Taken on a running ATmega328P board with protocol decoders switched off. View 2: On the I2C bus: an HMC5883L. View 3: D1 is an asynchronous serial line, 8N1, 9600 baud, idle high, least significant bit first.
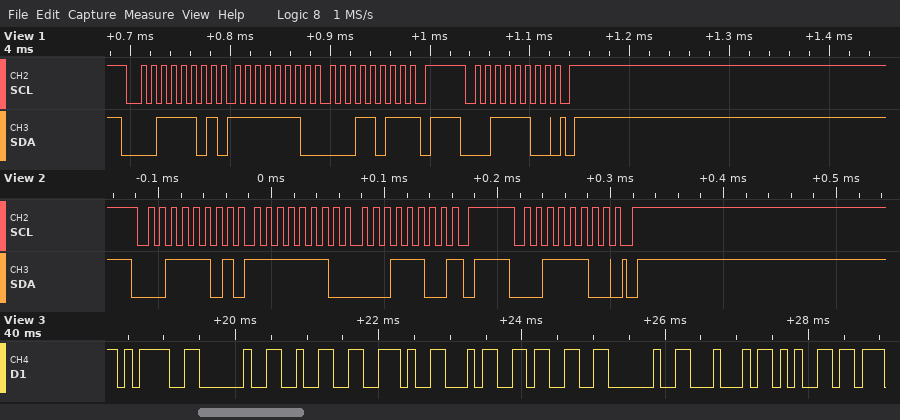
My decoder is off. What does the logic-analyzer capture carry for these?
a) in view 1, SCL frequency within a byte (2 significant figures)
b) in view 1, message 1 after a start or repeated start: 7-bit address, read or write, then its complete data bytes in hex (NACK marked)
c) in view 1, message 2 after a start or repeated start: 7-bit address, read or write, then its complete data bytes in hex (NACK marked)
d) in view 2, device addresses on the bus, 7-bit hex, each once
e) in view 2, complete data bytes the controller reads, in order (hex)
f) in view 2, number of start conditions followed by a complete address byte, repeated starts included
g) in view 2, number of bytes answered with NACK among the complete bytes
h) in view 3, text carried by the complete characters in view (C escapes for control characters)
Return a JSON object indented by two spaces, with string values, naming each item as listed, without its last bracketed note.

{
  "in view 1, SCL frequency within a byte": "100 kHz",
  "in view 1, message 1 after a start or repeated start: 7-bit address, read or write, then its complete data bytes in hex": "0x1E read: FE 1B NACK",
  "in view 1, message 2 after a start or repeated start: 7-bit address, read or write, then its complete data bytes in hex": "0x1E write",
  "in view 2, device addresses on the bus, 7-bit hex, each once": "0x1E",
  "in view 2, complete data bytes the controller reads, in order": "FE 1C",
  "in view 2, number of start conditions followed by a complete address byte, repeated starts included": "2",
  "in view 2, number of bytes answered with NACK among the complete bytes": "1",
  "in view 3, text carried by the complete characters in view": "\"= 2.43 De\""
}
